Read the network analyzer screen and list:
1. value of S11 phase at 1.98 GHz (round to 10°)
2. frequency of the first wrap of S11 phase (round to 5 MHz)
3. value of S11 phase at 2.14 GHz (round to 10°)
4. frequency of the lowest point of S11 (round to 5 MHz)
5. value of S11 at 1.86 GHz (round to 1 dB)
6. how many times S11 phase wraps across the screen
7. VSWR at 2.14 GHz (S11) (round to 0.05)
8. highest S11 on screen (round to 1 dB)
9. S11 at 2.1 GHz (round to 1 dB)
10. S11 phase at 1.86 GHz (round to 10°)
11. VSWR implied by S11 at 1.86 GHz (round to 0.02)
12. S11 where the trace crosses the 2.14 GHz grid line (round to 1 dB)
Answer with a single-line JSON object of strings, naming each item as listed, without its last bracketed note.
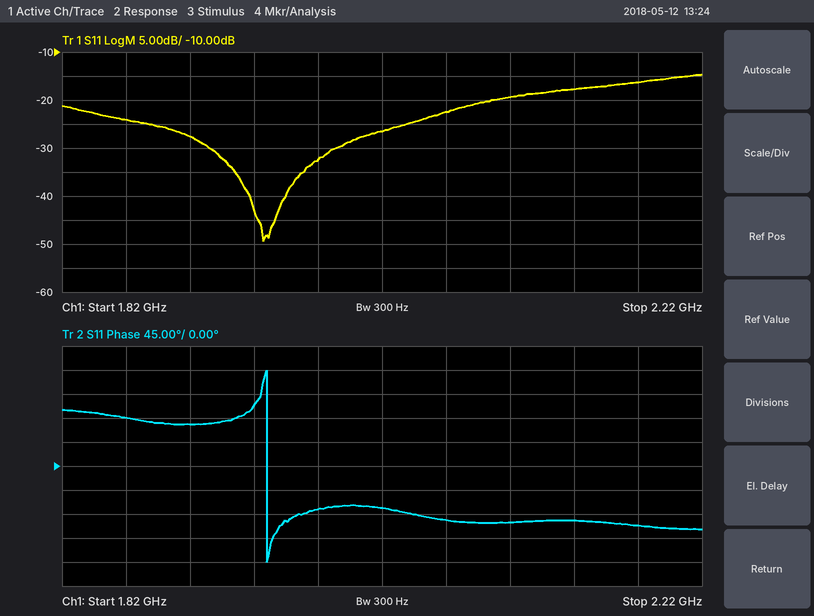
{"value of S11 phase at 1.98 GHz": "-80°", "frequency of the first wrap of S11 phase": "1.950 GHz", "value of S11 phase at 2.14 GHz": "-100°", "frequency of the lowest point of S11": "1.945 GHz", "value of S11 at 1.86 GHz": "-24 dB", "how many times S11 phase wraps across the screen": "1", "VSWR at 2.14 GHz (S11)": "1.30", "highest S11 on screen": "-15 dB", "S11 at 2.1 GHz": "-19 dB", "S11 phase at 1.86 GHz": "90°", "VSWR implied by S11 at 1.86 GHz": "1.14", "S11 where the trace crosses the 2.14 GHz grid line": "-18 dB"}
